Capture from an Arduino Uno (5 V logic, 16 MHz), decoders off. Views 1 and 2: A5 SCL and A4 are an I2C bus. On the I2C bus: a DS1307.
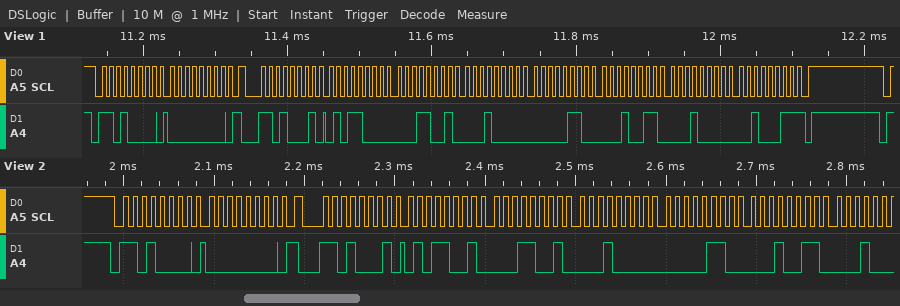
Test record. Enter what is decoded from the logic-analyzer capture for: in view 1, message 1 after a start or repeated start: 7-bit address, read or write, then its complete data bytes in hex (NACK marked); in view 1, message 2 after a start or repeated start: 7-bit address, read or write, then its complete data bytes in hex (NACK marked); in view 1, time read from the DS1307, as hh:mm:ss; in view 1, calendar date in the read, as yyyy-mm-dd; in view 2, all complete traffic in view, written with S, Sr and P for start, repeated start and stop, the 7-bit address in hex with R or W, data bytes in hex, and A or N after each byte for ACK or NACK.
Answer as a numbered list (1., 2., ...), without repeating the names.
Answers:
1. 0x68 write: 00
2. 0x68 read: 58 19 10 06 13 10 23 NACK
3. 10:19:58
4. 2023-10-13
5. S 68W A 00 A Sr 68R A 59 A 19 A 10 A 06 A 13 A
